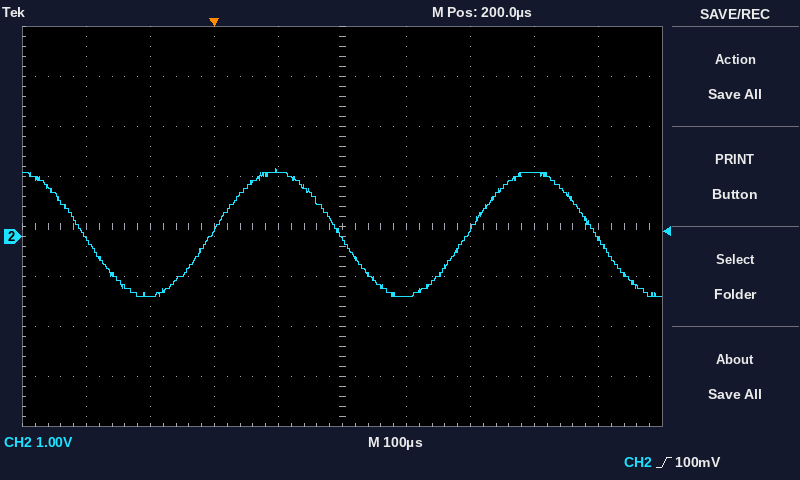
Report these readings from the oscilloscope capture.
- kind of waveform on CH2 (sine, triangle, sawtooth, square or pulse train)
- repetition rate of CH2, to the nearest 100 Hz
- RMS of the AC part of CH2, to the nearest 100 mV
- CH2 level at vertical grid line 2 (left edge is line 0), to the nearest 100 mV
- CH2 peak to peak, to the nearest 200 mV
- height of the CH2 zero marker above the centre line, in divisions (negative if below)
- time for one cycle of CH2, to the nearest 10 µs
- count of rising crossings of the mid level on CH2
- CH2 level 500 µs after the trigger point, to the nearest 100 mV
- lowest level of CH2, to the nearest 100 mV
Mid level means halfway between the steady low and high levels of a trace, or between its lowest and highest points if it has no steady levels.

sine
2.5 kHz
900 mV
-1.2 V
2.6 V
-0.2 div
400 µs
2
1.3 V
-1.2 V
